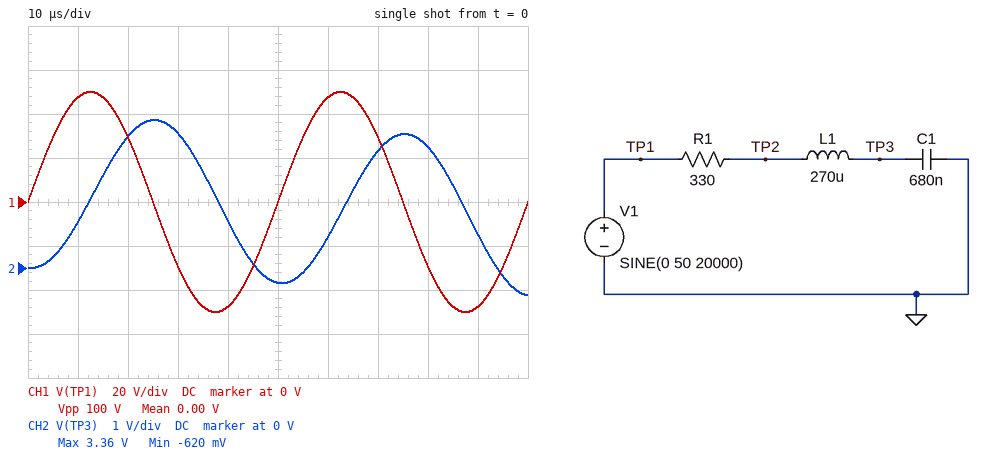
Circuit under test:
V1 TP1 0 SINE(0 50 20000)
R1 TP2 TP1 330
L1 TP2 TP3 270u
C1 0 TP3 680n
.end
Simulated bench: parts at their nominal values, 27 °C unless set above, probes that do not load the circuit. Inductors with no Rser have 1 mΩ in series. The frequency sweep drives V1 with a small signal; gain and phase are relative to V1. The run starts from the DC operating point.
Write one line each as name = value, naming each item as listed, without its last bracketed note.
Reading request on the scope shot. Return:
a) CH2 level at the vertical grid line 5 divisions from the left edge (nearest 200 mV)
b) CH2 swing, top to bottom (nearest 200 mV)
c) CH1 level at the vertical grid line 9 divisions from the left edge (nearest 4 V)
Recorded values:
CH2 level at the vertical grid line 5 divisions from the left edge = -400 mV
CH2 swing, top to bottom = 4.0 V
CH1 level at the vertical grid line 9 divisions from the left edge = -48 V
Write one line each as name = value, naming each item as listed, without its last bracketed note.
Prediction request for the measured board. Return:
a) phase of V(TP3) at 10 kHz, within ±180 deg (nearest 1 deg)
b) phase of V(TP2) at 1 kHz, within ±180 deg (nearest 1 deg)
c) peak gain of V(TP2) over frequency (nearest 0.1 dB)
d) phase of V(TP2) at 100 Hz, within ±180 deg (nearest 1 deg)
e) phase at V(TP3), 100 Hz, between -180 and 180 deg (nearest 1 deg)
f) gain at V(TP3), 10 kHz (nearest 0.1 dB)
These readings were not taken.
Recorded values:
phase of V(TP3) at 10 kHz, within ±180 deg = -89 deg
phase of V(TP2) at 1 kHz, within ±180 deg = -55 deg
peak gain of V(TP2) over frequency = 0 dB
phase of V(TP2) at 100 Hz, within ±180 deg = -8 deg
phase at V(TP3), 100 Hz, between -180 and 180 deg = -8 deg
gain at V(TP3), 10 kHz = -23.0 dB
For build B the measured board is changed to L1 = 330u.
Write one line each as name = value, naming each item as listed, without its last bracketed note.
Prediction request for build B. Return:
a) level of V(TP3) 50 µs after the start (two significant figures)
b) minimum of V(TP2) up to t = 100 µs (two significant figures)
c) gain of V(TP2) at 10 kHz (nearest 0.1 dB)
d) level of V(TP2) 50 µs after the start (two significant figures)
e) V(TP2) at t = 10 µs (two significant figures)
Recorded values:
level of V(TP3) 50 µs after the start = -330 mV
minimum of V(TP2) up to t = 100 µs = -3.2 V
gain of V(TP2) at 10 kHz = -41.8 dB
level of V(TP2) 50 µs after the start = 5.9 V
V(TP2) at t = 10 µs = 3.5 V
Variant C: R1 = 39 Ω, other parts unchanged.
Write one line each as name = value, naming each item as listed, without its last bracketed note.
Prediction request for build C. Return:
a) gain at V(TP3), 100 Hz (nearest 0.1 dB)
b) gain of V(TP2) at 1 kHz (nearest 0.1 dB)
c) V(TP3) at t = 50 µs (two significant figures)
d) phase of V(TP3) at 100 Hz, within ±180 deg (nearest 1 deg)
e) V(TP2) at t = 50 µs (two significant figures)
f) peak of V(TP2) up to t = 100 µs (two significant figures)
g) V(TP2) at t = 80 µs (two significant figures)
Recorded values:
gain at V(TP3), 100 Hz = 0 dB
gain of V(TP2) at 1 kHz = -0.1 dB
V(TP3) at t = 50 µs = -9.1 V
phase of V(TP3) at 100 Hz, within ±180 deg = -1 deg
V(TP2) at t = 50 µs = 25 V
peak of V(TP2) up to t = 100 µs = 28 V
V(TP2) at t = 80 µs = -24 V
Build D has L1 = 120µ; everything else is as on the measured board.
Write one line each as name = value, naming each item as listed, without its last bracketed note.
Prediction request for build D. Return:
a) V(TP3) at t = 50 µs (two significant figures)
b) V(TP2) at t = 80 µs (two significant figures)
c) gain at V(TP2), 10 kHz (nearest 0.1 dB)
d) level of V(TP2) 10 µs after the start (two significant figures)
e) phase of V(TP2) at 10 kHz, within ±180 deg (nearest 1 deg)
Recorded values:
V(TP3) at t = 50 µs = -350 mV
V(TP2) at t = 80 µs = 830 mV
gain at V(TP2), 10 kHz = -26.4 dB
level of V(TP2) 10 µs after the start = 1.9 V
phase of V(TP2) at 10 kHz, within ±180 deg = -87 deg
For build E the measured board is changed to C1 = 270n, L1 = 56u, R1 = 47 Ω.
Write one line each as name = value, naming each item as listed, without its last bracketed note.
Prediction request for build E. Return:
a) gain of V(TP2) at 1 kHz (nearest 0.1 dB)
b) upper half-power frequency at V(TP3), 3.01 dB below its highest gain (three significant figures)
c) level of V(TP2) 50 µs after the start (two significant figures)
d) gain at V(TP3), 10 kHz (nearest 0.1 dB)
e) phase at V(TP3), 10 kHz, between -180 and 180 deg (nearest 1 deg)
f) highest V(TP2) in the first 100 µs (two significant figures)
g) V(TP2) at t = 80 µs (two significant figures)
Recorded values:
gain of V(TP2) at 1 kHz = 0 dB
upper half-power frequency at V(TP3), 3.01 dB below its highest gain = 13.8 kHz
level of V(TP2) 50 µs after the start = -19 V
gain at V(TP3), 10 kHz = -1.8 dB
phase at V(TP3), 10 kHz, between -180 and 180 deg = -40 deg
highest V(TP2) in the first 100 µs = 26 V
V(TP2) at t = 80 µs = 10 V
